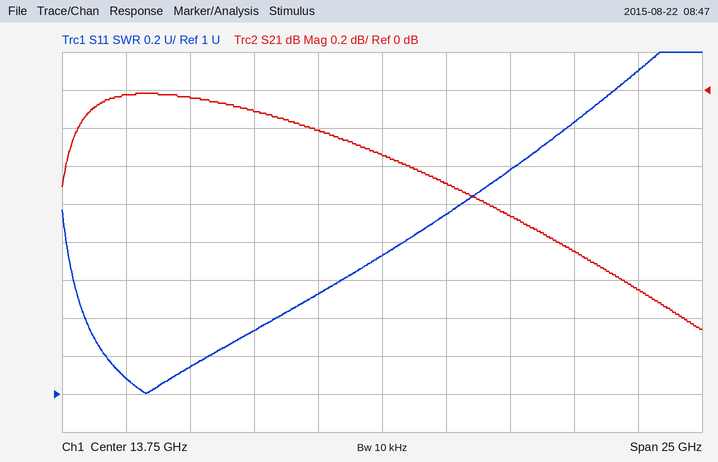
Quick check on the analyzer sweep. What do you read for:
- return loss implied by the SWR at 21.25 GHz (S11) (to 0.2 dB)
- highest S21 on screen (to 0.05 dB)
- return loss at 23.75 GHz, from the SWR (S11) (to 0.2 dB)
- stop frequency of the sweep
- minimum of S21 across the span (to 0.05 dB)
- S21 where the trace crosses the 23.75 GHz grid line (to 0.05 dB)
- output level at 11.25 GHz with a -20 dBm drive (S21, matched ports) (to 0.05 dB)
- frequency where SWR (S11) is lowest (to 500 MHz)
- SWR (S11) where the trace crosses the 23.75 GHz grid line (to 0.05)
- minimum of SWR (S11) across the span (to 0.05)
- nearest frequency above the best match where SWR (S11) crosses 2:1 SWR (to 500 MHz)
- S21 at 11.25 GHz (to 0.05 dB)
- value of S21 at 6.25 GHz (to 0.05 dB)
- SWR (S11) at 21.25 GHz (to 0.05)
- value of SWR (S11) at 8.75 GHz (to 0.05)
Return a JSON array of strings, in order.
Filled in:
["7.6 dB", "0.00 dB", "6.8 dB", "26.25 GHz", "-1.25 dB", "-1.05 dB", "-20.20 dBm", "4.5 GHz", "2.70", "1.00", "17.0 GHz", "-0.20 dB", "-0.05 dB", "2.45", "1.35"]
